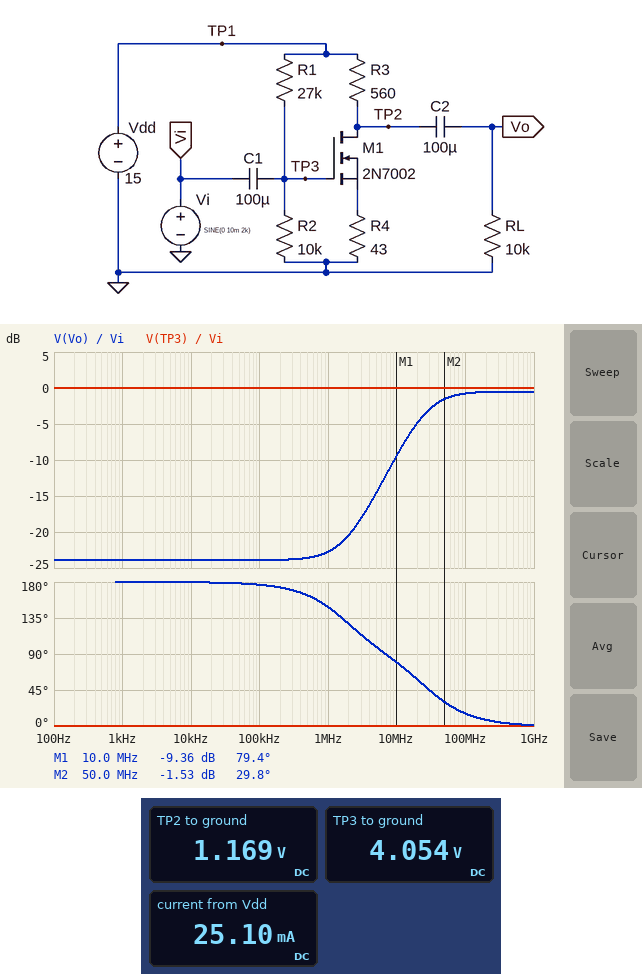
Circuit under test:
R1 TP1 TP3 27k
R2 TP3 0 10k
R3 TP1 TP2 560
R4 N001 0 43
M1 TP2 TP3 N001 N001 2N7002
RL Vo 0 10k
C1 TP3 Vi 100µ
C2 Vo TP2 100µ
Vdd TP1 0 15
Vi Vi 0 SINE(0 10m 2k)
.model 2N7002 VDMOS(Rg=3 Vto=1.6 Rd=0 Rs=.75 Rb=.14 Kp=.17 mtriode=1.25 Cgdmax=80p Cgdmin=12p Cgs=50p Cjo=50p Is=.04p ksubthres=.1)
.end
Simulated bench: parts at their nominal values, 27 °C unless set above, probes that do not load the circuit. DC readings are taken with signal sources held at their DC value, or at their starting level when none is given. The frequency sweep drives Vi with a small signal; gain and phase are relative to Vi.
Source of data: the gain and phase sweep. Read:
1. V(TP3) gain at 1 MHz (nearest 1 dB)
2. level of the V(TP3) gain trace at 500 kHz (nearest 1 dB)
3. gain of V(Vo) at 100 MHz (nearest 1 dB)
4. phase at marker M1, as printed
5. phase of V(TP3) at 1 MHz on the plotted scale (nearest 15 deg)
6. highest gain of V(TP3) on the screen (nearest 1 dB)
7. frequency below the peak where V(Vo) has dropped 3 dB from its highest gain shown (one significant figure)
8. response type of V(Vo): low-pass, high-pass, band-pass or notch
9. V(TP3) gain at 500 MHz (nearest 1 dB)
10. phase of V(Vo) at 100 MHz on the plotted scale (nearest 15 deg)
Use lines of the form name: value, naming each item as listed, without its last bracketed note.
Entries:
V(TP3) gain at 1 MHz: 0 dB
level of the V(TP3) gain trace at 500 kHz: 0 dB
gain of V(Vo) at 100 MHz: -1 dB
phase at marker M1, as printed: 79.4 deg
phase of V(TP3) at 1 MHz on the plotted scale: 0 deg
highest gain of V(TP3) on the screen: 0 dB
frequency below the peak where V(Vo) has dropped 3 dB from its highest gain shown: 30 MHz
response type of V(Vo): low-pass, high-pass, band-pass or notch: high-pass
V(TP3) gain at 500 MHz: 0 dB
phase of V(Vo) at 100 MHz on the plotted scale: 15 deg
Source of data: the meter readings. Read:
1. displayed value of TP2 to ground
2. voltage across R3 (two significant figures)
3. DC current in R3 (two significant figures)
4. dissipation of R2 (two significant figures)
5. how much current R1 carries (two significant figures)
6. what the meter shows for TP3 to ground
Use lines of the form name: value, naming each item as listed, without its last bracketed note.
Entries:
displayed value of TP2 to ground: 1.169 V
voltage across R3: 14 V
DC current in R3: 25 mA
dissipation of R2: 1.6 mW
how much current R1 carries: 410 µA
what the meter shows for TP3 to ground: 4.054 V
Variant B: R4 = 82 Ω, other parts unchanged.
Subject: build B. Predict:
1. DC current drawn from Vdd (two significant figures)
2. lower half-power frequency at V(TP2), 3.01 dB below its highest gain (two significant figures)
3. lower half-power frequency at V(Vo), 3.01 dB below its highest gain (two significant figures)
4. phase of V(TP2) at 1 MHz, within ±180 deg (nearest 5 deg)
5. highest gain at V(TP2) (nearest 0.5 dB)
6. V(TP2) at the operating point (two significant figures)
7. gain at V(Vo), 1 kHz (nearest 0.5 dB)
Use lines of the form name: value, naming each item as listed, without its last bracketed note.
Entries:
DC current drawn from Vdd: 23 mA
lower half-power frequency at V(TP2), 3.01 dB below its highest gain: 240 mHz
lower half-power frequency at V(Vo), 3.01 dB below its highest gain: 320 mHz
phase of V(TP2) at 1 MHz, within ±180 deg: 170 deg
highest gain at V(TP2): 0 dB
V(TP2) at the operating point: 2.2 V
gain at V(Vo), 1 kHz: -0.5 dB
